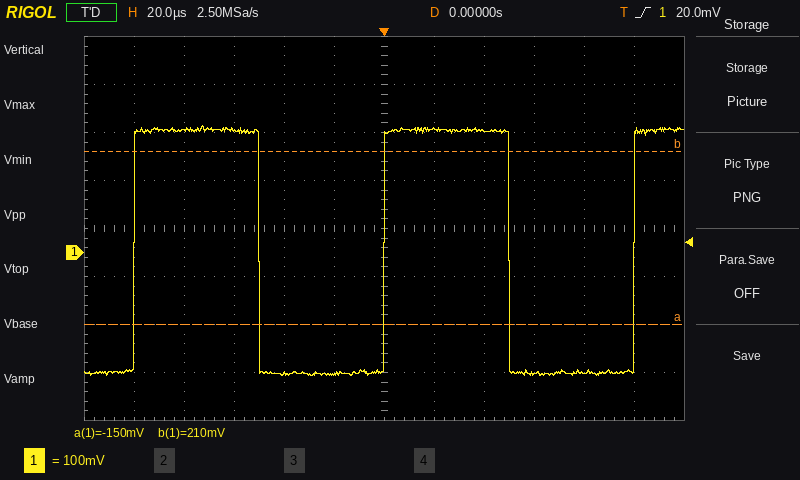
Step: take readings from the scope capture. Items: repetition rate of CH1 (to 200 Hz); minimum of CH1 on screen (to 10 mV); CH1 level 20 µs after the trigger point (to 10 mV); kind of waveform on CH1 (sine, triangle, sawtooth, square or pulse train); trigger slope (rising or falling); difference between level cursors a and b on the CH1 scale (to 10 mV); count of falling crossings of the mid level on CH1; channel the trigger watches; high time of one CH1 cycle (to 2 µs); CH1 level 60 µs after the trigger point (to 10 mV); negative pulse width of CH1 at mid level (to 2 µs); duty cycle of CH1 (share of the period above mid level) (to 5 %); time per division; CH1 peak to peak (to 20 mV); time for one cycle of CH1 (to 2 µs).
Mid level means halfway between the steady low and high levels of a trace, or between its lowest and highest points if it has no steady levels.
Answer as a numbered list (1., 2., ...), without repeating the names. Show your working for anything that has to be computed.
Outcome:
1. 1 / 100 µs ≈ 10.0 kHz
2. -260 mV
3. 260 mV
4. square
5. rising
6. 360 mV
7. 2
8. CH1
9. 50 µs
10. -250 mV
11. 50 µs
12. 50 µs / 100 µs ≈ 50 %
13. 20 µs
14. 520 mV
15. 100 µs
